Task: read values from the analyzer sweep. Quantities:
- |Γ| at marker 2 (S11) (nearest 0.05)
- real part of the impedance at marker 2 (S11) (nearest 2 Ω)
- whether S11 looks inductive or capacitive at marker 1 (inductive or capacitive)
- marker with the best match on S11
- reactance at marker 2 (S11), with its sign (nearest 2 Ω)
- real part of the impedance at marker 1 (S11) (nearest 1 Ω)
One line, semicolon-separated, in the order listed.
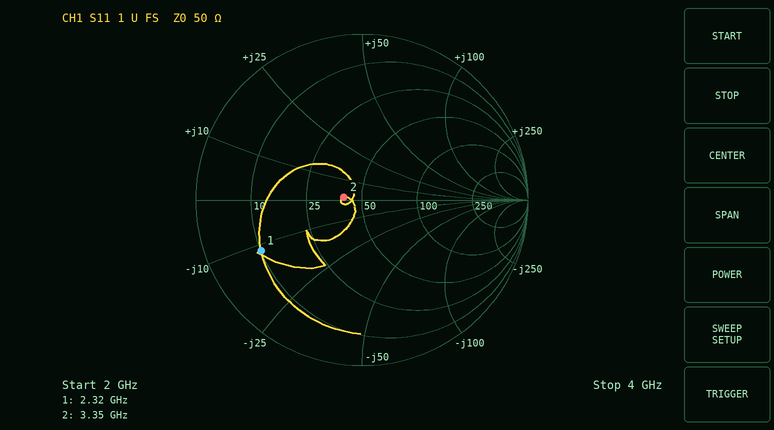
0.10; 40 Ω; capacitive; marker 2; +2 Ω; 10 Ω
